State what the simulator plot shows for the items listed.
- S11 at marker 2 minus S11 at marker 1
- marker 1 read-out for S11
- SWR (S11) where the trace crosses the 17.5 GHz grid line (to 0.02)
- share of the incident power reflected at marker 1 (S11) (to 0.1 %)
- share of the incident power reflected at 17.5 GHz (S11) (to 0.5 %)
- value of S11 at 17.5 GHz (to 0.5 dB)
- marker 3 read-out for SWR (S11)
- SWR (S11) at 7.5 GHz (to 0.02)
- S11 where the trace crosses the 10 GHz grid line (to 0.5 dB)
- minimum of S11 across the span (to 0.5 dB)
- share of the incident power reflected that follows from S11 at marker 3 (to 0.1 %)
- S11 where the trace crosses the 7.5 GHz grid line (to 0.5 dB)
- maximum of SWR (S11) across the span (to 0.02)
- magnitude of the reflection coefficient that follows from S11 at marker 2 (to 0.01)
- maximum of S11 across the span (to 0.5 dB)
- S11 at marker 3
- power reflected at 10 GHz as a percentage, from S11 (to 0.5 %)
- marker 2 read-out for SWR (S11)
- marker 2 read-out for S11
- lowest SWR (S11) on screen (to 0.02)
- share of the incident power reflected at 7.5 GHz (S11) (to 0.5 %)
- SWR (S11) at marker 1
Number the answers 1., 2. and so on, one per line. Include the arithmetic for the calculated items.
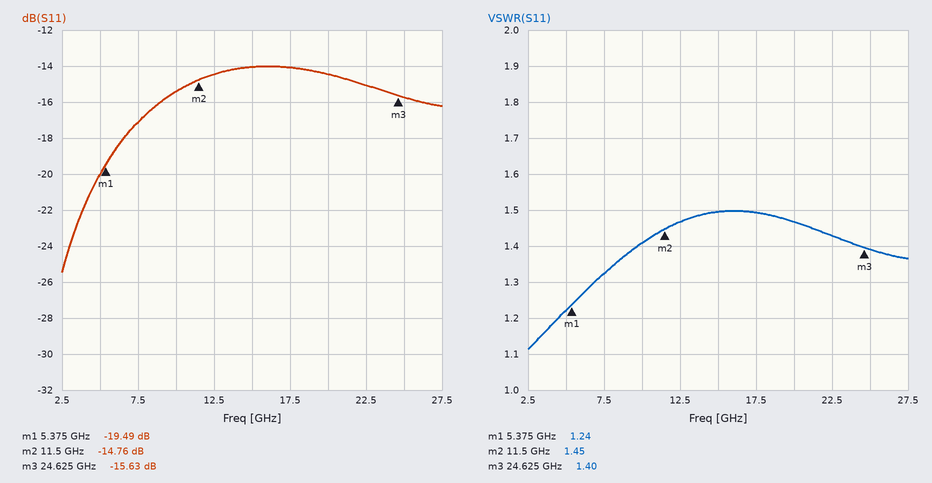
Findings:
1. -14.76 − (-19.49) = 4.73 dB
2. -19.49 dB
3. 1.50
4. 10^(-19.49/10) ≈ 1.1 %
5. 10^(-14/10) ≈ 4.0 %
6. -14.0 dB
7. 1.40
8. 1.32
9. -15.5 dB
10. -25.5 dB
11. 10^(-15.63/10) ≈ 2.7 %
12. -17.0 dB
13. 1.50
14. 10^(-14.76/20) ≈ 0.18
15. -14.0 dB
16. -15.63 dB
17. 10^(-15.5/10) ≈ 2.82 %, so 3.0 % to the nearest 0.5 %
18. 1.45
19. -14.76 dB
20. 1.12
21. 10^(-17/10) ≈ 2.0 %
22. 1.24
